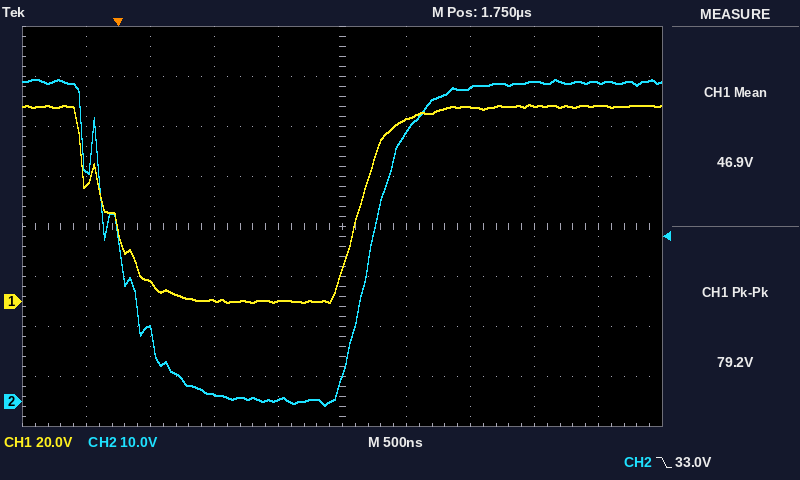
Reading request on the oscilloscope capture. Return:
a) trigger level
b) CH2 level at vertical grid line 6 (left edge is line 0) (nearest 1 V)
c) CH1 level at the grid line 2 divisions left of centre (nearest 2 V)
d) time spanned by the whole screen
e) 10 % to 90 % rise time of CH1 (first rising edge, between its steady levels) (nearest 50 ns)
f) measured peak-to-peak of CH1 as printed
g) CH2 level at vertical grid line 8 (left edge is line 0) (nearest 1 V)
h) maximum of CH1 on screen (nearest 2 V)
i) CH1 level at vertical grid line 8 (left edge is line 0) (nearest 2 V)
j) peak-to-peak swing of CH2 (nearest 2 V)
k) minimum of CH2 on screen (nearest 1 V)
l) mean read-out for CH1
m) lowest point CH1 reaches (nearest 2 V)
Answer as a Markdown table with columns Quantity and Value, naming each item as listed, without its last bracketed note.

| Quantity | Value |
|---|---|
| trigger level | 33.0 V |
| CH2 level at vertical grid line 6 (left edge is line 0) | 54 V |
| CH1 level at the grid line 2 divisions left of centre | 0 V |
| time spanned by the whole screen | 5 µs |
| 10 % to 90 % rise time of CH1 (first rising edge, between its steady levels) | 450 ns |
| measured peak-to-peak of CH1 as printed | 79.2 V |
| CH2 level at vertical grid line 8 (left edge is line 0) | 64 V |
| maximum of CH1 on screen | 78 V |
| CH1 level at vertical grid line 8 (left edge is line 0) | 78 V |
| peak-to-peak swing of CH2 | 66 V |
| minimum of CH2 on screen | -1 V |
| mean read-out for CH1 | 46.9 V |
| lowest point CH1 reaches | 0 V |
